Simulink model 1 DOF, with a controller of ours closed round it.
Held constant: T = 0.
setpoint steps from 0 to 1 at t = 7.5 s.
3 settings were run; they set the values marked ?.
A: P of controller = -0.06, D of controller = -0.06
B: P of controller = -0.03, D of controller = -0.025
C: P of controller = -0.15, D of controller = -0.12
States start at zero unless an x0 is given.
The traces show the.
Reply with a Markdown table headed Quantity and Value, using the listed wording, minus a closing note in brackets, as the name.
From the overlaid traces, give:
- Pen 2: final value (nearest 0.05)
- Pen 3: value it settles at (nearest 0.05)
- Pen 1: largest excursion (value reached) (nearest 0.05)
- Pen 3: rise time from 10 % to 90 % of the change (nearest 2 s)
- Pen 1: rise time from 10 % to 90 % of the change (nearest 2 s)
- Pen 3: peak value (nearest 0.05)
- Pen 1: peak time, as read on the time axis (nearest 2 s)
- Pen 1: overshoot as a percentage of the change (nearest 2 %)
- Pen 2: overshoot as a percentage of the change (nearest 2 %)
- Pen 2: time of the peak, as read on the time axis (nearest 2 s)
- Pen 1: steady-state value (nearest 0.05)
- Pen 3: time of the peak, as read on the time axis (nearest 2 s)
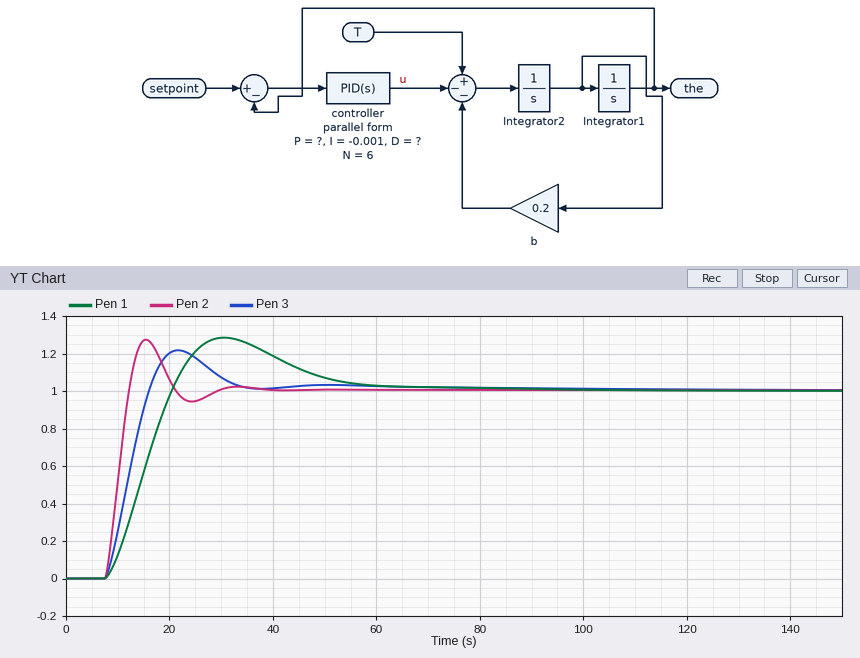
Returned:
| Quantity | Value |
|---|---|
| Pen 2: final value | 1.00 |
| Pen 3: value it settles at | 1.00 |
| Pen 1: largest excursion (value reached) | 1.30 |
| Pen 3: rise time from 10 % to 90 % of the change | 6 s |
| Pen 1: rise time from 10 % to 90 % of the change | 10 s |
| Pen 3: peak value | 1.20 |
| Pen 1: peak time, as read on the time axis | 30 s |
| Pen 1: overshoot as a percentage of the change | 28 % |
| Pen 2: overshoot as a percentage of the change | 28 % |
| Pen 2: time of the peak, as read on the time axis | 16 s |
| Pen 1: steady-state value | 1.00 |
| Pen 3: time of the peak, as read on the time axis | 22 s |
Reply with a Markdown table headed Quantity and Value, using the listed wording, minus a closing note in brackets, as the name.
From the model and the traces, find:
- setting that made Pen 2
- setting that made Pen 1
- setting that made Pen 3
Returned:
| Quantity | Value |
|---|---|
| setting that made Pen 2 | C |
| setting that made Pen 1 | B |
| setting that made Pen 3 | A |
